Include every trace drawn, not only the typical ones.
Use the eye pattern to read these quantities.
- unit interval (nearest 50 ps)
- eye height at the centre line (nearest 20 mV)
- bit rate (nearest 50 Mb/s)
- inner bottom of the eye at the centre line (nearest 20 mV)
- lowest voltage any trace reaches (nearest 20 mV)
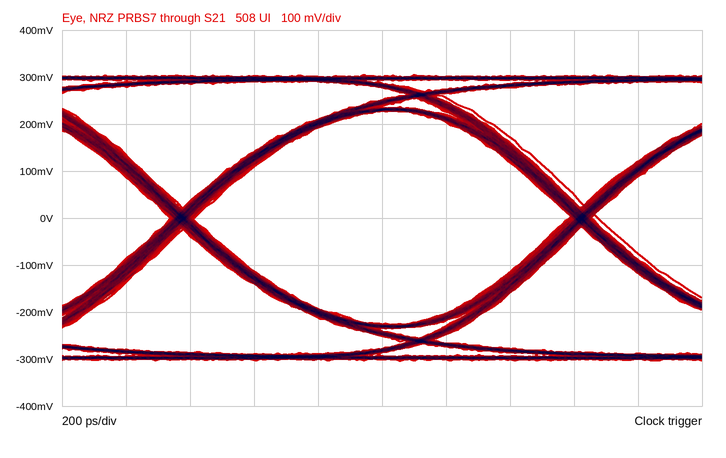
1.25 ns
460 mV
800 Mb/s
-220 mV
-300 mV
